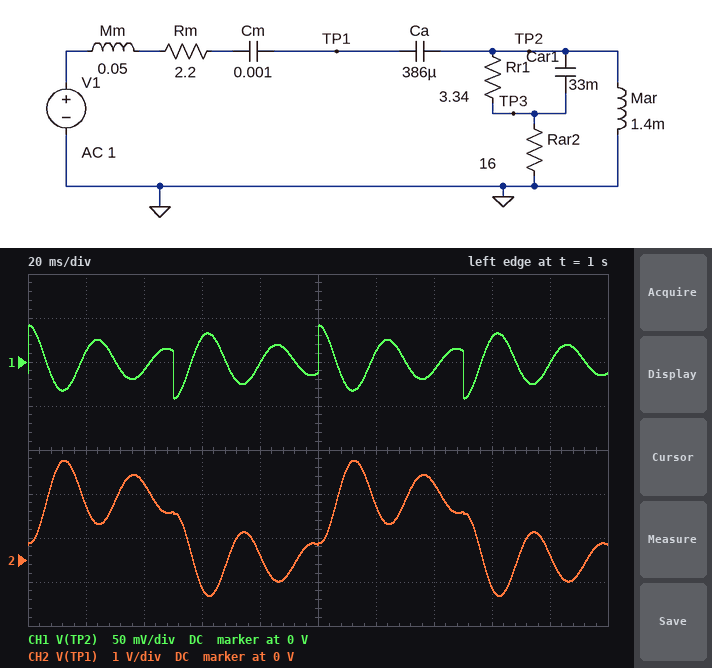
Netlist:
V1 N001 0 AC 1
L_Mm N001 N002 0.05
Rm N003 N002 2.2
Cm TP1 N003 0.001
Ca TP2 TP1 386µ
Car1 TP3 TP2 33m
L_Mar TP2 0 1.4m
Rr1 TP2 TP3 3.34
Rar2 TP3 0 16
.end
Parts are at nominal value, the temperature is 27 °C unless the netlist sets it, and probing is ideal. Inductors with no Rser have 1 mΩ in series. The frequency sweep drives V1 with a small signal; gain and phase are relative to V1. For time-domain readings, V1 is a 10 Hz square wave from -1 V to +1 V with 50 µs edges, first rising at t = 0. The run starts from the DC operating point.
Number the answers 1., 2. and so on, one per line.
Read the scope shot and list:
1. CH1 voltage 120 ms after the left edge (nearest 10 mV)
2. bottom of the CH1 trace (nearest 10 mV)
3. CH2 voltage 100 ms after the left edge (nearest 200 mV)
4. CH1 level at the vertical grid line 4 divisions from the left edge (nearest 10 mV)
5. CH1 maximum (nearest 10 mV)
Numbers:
1. 10 mV
2. -40 mV
3. 400 mV
4. 0 V
5. 40 mV
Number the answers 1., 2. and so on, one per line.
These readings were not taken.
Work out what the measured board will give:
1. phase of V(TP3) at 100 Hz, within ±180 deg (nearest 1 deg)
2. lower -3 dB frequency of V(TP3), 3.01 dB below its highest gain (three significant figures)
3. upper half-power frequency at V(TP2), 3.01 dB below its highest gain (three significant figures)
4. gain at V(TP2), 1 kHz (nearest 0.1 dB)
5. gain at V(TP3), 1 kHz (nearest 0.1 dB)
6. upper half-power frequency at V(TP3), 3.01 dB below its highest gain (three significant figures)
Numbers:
1. 2 deg
2. 39.2 Hz
3. 46.3 Hz
4. -32.4 dB
5. -32.4 dB
6. 46.3 Hz
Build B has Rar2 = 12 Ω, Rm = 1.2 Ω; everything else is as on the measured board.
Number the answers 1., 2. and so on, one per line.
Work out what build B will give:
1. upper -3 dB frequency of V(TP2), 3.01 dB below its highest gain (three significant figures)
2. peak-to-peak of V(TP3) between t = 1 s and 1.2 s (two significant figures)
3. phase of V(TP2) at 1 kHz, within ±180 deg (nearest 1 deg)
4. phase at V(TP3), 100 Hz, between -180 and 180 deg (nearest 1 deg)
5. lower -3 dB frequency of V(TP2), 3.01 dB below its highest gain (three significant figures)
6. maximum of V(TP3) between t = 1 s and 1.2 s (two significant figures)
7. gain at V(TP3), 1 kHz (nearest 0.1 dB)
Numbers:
1. 44.2 Hz
2. 73 mV
3. -35 deg
4. -1 deg
5. 40.4 Hz
6. 37 mV
7. -33.1 dB
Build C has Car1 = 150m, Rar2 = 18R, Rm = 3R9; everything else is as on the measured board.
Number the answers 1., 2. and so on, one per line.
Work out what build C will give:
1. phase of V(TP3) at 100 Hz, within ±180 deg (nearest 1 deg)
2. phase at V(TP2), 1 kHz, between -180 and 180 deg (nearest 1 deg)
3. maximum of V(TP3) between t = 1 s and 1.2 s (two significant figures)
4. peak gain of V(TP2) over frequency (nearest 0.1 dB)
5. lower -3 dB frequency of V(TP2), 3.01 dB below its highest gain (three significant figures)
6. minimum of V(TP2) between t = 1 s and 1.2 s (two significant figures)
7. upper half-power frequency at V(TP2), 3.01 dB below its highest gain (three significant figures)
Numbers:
1. 6 deg
2. -25 deg
3. 47 mV
4. -20.4 dB
5. 37.7 Hz
6. -47 mV
7. 51.2 Hz
